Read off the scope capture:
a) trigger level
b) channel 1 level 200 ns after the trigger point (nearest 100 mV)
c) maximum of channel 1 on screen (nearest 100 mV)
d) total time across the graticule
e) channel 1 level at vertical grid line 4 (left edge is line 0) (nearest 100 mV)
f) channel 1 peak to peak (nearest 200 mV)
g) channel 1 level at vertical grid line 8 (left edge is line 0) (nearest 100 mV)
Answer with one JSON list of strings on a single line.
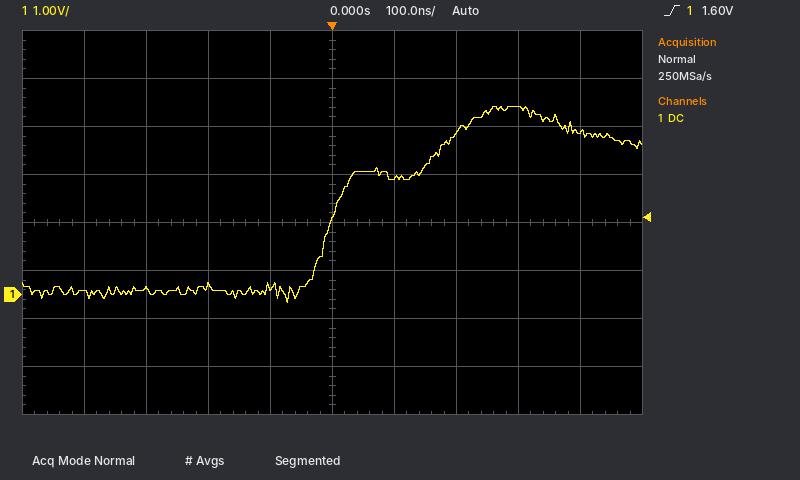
["1.60 V", "3.4 V", "3.9 V", "1 µs", "200 mV", "4.0 V", "3.9 V"]
